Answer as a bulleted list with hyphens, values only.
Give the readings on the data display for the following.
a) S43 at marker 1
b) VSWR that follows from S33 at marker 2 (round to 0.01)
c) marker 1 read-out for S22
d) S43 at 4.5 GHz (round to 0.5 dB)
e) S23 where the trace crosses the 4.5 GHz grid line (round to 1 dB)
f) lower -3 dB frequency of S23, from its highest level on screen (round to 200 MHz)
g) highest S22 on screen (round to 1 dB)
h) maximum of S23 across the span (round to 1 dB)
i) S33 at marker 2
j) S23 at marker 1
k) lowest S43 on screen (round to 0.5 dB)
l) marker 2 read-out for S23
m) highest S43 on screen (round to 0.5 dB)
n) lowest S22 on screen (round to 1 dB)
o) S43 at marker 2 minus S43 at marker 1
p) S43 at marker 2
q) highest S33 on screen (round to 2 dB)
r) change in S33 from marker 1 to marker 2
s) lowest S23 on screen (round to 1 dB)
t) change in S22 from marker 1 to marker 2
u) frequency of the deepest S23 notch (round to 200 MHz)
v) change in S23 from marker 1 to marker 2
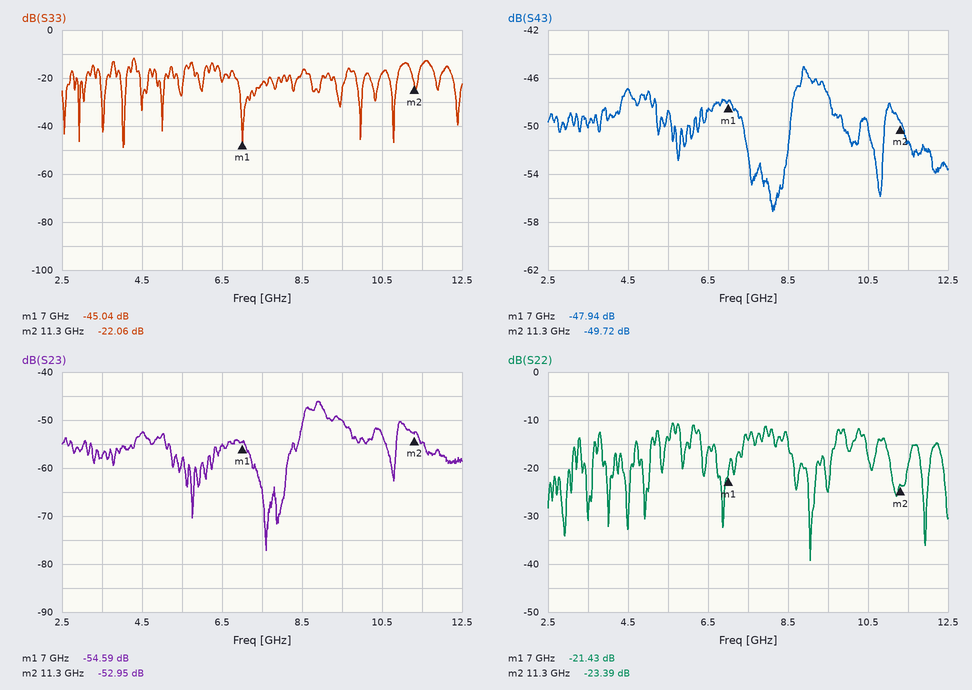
- -47.94 dB
- 1.17
- -21.43 dB
- -47.0 dB
- -53 dB
- 8.6 GHz
- -11 dB
- -46 dB
- -22.06 dB
- -54.59 dB
- -57.0 dB
- -52.95 dB
- -45.0 dB
- -39 dB
- -1.78 dB
- -49.72 dB
- -12 dB
- 22.98 dB
- -77 dB
- -1.96 dB
- 7.6 GHz
- 1.64 dB
